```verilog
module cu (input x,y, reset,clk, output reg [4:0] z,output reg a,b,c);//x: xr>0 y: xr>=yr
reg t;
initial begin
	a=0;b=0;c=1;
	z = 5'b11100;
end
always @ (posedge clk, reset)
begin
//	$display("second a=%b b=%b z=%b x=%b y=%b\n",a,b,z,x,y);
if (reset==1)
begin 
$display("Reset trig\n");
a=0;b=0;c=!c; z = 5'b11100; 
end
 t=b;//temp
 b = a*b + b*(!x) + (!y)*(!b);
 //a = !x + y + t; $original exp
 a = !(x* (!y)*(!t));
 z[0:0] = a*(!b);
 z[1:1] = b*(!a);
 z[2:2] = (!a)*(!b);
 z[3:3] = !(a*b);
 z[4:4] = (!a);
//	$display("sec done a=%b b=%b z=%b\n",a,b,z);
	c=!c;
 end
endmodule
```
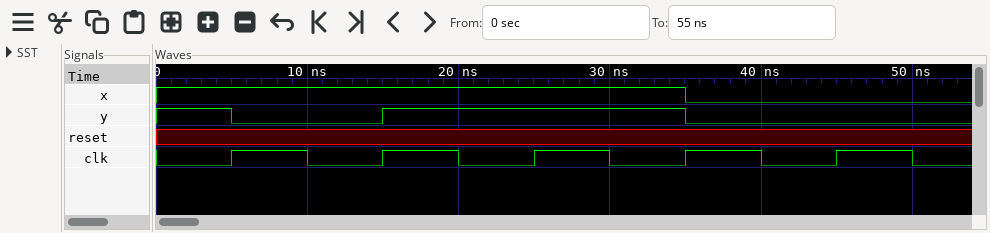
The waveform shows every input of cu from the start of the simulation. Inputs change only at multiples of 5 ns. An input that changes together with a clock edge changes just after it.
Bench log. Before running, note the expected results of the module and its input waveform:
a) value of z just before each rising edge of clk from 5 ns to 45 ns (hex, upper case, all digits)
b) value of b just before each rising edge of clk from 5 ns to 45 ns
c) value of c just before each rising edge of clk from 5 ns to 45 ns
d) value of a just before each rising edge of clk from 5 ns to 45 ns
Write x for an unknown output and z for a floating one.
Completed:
1C, 09, 1A, 09, 09
0 0 1 0 0
1 0 1 0 1
0 1 0 1 1
